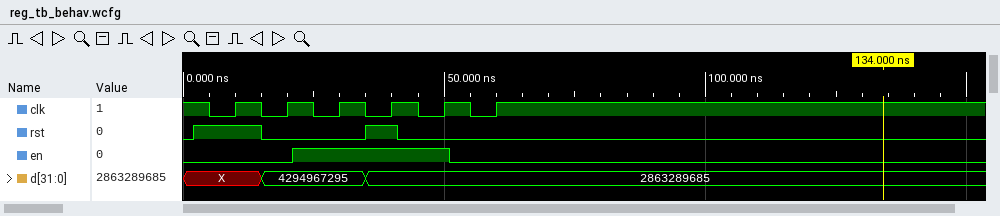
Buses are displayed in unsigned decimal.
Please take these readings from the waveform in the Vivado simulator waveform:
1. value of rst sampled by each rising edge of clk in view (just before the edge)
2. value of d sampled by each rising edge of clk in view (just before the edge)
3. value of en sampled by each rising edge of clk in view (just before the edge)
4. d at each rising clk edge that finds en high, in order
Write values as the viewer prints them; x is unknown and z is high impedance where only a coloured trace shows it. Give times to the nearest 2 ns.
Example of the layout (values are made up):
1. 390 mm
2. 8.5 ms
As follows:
1. 1 0 0 1 0 0
2. X, 4294967295, 4294967295, 2863289685, 2863289685, 2863289685
3. 0 0 1 1 1 0
4. 4294967295, 2863289685, 2863289685
